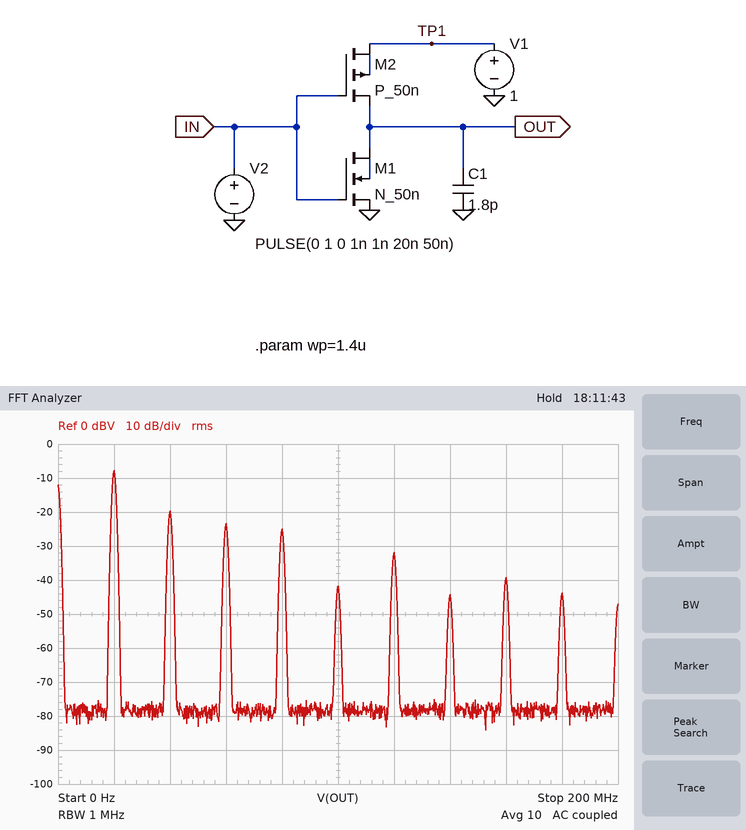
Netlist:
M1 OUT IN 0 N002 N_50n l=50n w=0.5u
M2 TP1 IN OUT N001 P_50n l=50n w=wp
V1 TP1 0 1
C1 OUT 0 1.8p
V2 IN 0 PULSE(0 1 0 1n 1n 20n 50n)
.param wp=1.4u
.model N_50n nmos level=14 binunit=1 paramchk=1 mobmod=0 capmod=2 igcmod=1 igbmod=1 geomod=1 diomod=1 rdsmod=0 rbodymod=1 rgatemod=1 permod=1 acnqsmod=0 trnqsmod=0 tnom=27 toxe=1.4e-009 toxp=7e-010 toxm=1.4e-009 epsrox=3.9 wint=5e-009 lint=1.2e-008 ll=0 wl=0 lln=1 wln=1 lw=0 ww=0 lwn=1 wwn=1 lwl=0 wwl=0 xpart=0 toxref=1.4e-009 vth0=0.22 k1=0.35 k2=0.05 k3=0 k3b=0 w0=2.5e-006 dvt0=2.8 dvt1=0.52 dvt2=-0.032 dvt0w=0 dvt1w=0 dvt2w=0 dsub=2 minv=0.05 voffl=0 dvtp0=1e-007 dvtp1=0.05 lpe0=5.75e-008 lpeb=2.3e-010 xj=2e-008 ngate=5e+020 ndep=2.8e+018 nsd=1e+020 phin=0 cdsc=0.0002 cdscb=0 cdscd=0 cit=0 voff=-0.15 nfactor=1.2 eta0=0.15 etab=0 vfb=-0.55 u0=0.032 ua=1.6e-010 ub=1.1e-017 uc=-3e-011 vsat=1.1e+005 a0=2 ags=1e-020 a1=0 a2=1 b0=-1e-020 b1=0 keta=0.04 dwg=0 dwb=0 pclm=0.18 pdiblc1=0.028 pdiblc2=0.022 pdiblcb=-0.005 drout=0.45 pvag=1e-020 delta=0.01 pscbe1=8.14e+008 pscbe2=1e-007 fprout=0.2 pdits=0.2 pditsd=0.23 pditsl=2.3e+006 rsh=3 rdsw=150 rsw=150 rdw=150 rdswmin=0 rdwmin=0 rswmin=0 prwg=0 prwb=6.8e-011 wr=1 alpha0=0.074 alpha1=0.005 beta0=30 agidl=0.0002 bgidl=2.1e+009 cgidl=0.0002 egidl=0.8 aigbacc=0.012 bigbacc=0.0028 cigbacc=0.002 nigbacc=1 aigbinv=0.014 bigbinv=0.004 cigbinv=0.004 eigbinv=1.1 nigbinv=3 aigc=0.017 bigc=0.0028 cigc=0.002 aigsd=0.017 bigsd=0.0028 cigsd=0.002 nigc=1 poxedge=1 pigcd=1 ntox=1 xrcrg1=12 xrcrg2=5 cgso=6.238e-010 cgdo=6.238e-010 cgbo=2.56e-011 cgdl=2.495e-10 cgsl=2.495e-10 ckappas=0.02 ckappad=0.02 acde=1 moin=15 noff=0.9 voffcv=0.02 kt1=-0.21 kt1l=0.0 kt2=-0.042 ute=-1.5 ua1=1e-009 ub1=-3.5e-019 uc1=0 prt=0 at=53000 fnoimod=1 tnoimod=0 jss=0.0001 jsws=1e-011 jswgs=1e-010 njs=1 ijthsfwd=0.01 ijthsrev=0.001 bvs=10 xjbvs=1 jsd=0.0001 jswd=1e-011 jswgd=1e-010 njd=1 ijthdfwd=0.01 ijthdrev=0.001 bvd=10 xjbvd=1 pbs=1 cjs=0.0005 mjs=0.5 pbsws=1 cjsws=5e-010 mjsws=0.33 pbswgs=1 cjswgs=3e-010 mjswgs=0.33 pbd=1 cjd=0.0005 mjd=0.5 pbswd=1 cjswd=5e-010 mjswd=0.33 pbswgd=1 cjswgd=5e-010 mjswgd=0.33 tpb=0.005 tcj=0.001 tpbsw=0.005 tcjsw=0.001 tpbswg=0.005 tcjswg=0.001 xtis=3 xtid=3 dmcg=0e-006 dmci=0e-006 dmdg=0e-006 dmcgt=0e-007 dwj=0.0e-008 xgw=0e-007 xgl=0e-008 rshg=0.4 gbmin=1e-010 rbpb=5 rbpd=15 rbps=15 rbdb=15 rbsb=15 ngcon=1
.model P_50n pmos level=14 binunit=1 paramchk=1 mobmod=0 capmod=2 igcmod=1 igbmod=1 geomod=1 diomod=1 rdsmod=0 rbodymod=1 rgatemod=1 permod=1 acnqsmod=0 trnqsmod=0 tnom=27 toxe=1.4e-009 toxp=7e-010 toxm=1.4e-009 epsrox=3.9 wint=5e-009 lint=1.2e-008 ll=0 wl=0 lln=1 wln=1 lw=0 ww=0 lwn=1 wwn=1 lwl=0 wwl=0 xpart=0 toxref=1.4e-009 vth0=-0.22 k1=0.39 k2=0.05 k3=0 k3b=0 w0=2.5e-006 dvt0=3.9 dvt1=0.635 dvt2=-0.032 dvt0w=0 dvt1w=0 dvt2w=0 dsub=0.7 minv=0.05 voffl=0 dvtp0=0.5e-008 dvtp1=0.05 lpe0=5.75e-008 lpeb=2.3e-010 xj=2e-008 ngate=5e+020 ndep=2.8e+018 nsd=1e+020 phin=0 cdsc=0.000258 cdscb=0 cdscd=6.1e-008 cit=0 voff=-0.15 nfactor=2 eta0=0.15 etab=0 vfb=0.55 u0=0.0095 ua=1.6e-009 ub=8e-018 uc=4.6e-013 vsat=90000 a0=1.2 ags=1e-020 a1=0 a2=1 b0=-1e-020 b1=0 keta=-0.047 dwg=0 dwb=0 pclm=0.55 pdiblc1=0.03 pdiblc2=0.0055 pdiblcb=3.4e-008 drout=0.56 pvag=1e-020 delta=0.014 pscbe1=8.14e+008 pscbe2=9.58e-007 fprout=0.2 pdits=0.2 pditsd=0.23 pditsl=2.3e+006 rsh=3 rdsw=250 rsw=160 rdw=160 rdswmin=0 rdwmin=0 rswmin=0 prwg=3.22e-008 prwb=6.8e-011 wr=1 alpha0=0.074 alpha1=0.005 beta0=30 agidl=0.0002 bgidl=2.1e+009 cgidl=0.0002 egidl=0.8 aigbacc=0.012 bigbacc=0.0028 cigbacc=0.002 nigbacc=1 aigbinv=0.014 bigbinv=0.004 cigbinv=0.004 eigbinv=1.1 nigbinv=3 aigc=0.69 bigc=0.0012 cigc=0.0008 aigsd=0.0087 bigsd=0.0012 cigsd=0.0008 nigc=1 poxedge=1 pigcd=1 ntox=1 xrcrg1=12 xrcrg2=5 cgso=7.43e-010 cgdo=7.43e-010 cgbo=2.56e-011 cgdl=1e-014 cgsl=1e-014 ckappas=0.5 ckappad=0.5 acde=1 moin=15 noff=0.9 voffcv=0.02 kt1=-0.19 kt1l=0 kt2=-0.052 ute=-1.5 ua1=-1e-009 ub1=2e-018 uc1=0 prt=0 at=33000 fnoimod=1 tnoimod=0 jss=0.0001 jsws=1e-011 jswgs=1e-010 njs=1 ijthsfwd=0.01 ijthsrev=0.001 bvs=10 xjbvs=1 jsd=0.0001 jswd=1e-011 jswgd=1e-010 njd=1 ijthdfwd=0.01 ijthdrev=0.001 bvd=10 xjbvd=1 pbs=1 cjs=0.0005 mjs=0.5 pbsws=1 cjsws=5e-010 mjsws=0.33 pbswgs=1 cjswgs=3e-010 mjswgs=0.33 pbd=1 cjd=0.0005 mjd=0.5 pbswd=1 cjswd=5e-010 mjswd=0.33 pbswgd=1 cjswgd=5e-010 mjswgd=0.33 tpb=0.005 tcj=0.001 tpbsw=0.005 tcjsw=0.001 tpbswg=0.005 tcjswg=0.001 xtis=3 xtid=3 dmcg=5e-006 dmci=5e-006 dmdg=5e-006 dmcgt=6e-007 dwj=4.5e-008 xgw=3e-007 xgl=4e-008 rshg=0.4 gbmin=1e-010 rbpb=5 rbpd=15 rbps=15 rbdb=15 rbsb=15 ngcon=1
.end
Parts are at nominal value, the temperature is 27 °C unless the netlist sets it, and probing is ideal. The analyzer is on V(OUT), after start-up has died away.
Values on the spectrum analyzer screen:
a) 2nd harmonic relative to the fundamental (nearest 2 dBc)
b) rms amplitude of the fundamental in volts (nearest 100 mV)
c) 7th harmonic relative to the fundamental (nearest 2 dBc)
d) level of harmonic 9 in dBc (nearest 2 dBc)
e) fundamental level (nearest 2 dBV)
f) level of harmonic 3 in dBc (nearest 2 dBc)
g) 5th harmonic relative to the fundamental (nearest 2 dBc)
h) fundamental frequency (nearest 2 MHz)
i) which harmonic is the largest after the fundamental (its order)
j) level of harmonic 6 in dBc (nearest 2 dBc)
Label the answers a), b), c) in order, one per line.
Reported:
a) -12 dBc
b) 400 mV
c) -36 dBc
d) -36 dBc
e) -8 dBV
f) -16 dBc
g) -34 dBc
h) 20 MHz
i) 2
j) -24 dBc
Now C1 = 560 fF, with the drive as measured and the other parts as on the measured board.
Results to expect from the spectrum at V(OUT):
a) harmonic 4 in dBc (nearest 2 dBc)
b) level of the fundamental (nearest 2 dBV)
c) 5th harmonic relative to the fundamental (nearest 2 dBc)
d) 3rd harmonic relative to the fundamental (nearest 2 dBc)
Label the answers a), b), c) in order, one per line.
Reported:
a) -14 dBc
b) -8 dBV
c) -26 dBc
d) -12 dBc
